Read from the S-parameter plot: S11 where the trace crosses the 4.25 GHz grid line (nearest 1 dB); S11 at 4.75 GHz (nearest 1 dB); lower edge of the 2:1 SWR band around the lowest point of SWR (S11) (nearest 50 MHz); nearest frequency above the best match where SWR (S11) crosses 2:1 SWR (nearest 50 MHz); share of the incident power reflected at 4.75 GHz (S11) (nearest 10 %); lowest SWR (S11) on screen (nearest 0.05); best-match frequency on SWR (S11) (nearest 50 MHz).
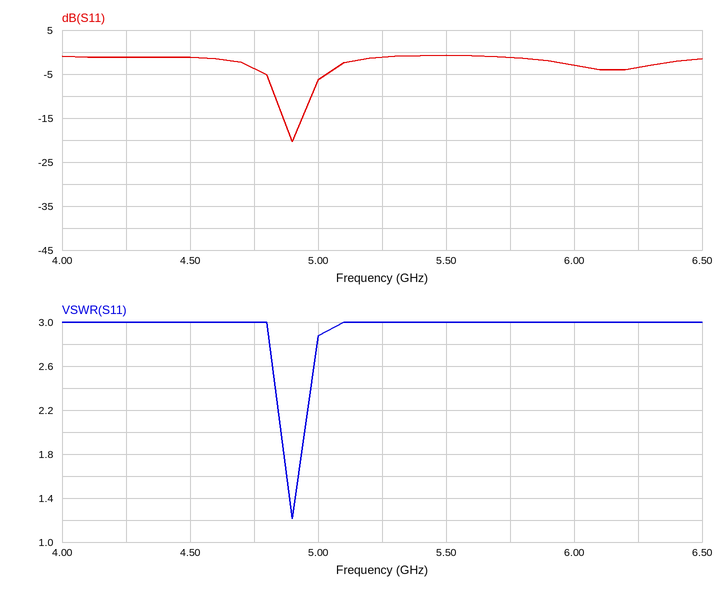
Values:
-1 dB
-4 dB
4.85 GHz
4.95 GHz
40 %
1.20
4.90 GHz
